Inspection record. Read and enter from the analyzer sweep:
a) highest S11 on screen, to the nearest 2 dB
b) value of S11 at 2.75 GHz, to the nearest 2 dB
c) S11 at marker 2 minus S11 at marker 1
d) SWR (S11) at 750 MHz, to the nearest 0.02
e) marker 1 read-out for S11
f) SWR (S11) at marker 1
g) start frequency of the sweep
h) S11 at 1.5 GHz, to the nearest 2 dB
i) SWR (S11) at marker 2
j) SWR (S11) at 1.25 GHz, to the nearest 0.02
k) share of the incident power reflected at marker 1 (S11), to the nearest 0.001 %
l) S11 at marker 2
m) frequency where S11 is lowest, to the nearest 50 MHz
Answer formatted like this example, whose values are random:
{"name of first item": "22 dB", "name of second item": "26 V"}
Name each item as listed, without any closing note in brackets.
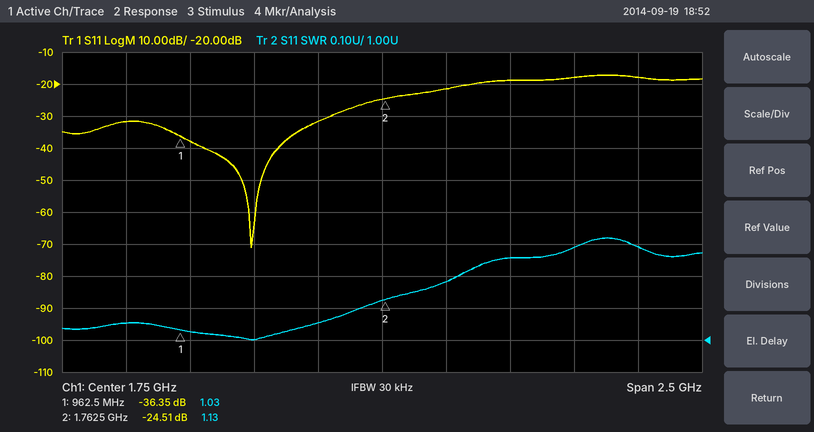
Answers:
{"highest S11 on screen, to the nearest 2 dB": "-18 dB", "value of S11 at 2.75 GHz, to the nearest 2 dB": "-18 dB", "S11 at marker 2 minus S11 at marker 1": "11.84 dB", "SWR (S11) at 750 MHz, to the nearest 0.02": "1.06", "marker 1 read-out for S11": "-36.35 dB", "SWR (S11) at marker 1": "1.03", "start frequency of the sweep": "500 MHz", "S11 at 1.5 GHz, to the nearest 2 dB": "-32 dB", "SWR (S11) at marker 2": "1.13", "SWR (S11) at 1.25 GHz, to the nearest 0.02": "1.00", "share of the incident power reflected at marker 1 (S11), to the nearest 0.001 %": "0.023 %", "S11 at marker 2": "-24.51 dB", "frequency where S11 is lowest, to the nearest 50 MHz": "1.25 GHz"}
